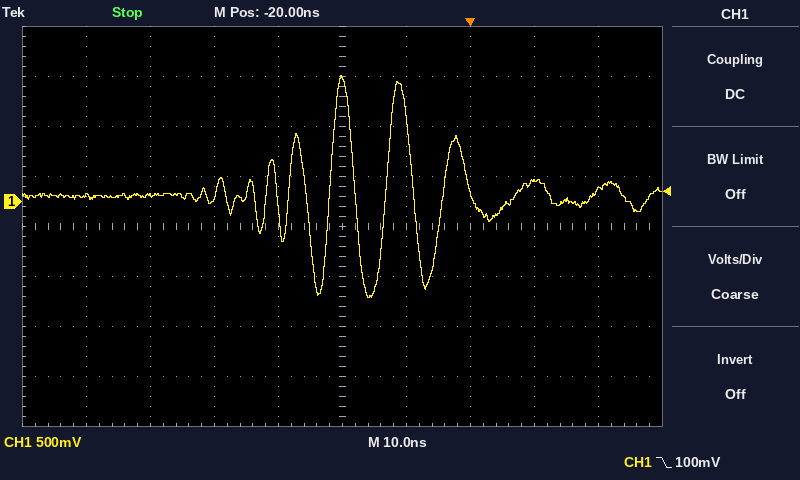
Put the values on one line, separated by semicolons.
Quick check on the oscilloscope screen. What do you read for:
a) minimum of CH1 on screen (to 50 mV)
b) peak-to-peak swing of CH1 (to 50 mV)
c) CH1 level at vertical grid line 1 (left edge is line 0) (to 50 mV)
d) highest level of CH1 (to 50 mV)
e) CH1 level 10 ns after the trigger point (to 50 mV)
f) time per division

-950 mV; 2.20 V; 50 mV; 1.25 V; 200 mV; 10 ns
